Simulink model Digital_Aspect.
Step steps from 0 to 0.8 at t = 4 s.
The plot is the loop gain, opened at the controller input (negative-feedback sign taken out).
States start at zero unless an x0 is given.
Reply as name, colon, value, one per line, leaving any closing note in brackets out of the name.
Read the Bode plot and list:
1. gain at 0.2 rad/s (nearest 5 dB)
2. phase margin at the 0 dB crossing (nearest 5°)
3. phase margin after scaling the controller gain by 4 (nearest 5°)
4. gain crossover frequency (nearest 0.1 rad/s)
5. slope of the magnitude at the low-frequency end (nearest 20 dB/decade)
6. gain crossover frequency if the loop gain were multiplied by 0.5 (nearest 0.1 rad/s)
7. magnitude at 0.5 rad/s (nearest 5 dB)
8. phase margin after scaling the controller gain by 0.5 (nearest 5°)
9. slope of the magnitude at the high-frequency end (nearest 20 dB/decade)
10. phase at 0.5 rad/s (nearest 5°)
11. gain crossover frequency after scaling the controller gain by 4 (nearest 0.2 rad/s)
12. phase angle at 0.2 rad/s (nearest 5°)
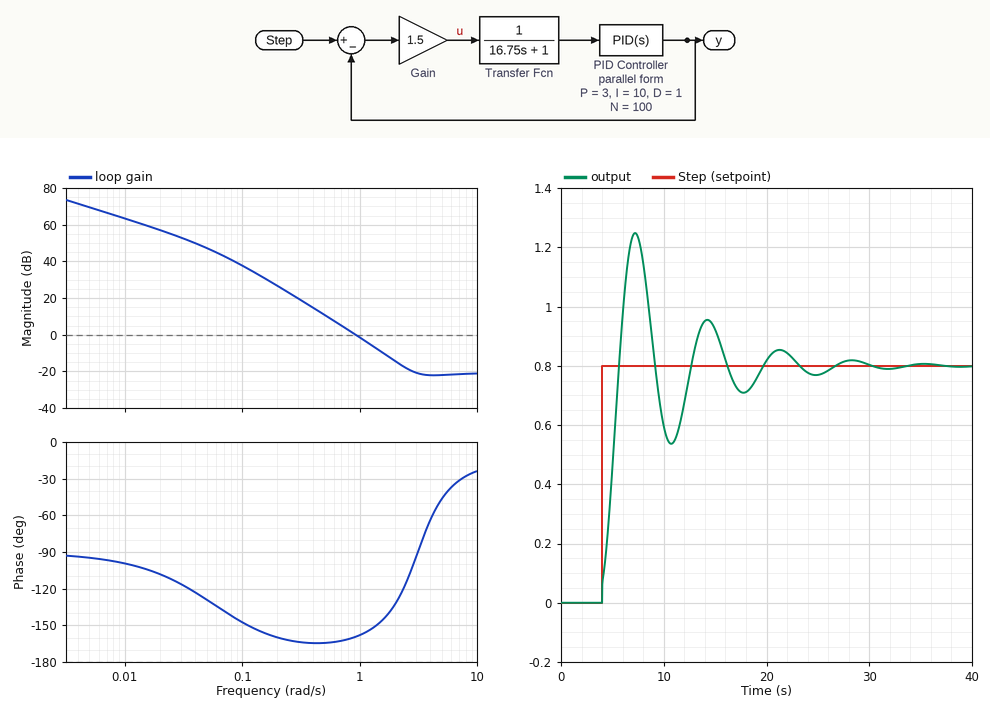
gain at 0.2 rad/s: 25 dB
phase margin at the 0 dB crossing: 20°
phase margin after scaling the controller gain by 4: 40°
gain crossover frequency: 0.9 rad/s
slope of the magnitude at the low-frequency end: -20 dB/decade
gain crossover frequency if the loop gain were multiplied by 0.5: 0.7 rad/s
magnitude at 0.5 rad/s: 10 dB
phase margin after scaling the controller gain by 0.5: 15°
slope of the magnitude at the high-frequency end: 0 dB/decade
phase at 0.5 rad/s: -165°
gain crossover frequency after scaling the controller gain by 4: 1.8 rad/s
phase angle at 0.2 rad/s: -160°
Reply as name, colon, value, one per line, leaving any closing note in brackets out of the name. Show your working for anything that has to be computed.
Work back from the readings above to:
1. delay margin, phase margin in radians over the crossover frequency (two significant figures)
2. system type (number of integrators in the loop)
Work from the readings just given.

delay margin, phase margin in radians over the crossover frequency: 20 × π / 180 / 0.9 = 0.39 s
system type: 1
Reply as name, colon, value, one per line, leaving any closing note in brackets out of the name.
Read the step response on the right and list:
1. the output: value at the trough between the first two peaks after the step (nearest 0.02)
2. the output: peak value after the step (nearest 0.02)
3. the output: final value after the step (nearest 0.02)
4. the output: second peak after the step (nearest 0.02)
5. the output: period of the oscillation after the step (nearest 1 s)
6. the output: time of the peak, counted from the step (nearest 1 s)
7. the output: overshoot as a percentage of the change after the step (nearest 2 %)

the output: value at the trough between the first two peaks after the step: 0.54
the output: peak value after the step: 1.24
the output: final value after the step: 0.80
the output: second peak after the step: 0.96
the output: period of the oscillation after the step: 7 s
the output: time of the peak, counted from the step: 3 s
the output: overshoot as a percentage of the change after the step: 56 %
